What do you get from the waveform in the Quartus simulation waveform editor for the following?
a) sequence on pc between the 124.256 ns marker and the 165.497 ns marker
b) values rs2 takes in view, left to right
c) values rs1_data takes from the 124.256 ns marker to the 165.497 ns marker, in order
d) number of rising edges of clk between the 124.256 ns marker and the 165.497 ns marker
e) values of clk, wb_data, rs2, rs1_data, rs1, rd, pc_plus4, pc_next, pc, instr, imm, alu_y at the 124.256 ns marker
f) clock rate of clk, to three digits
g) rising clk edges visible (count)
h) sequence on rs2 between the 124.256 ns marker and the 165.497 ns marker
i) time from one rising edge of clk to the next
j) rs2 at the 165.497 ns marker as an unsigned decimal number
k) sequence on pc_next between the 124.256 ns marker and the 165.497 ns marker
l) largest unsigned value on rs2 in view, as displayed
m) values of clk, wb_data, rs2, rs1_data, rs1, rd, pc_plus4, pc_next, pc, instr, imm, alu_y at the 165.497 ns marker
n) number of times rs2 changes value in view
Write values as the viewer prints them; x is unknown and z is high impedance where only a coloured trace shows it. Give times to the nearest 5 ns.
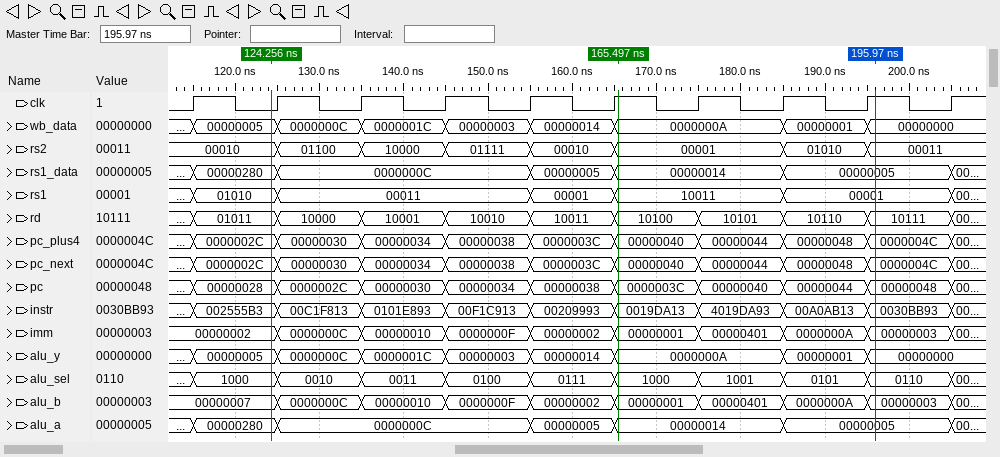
00000028, 0000002C, 00000030, 00000034, 00000038, 0000003C
00010, 01100, 10000, 01111, 00010, 00001, 01010, 00011
00000280, 0000000C, 00000005, 00000014
5
clk=0, wb_data=00000005, rs2=00010, rs1_data=00000280, rs1=01010, rd=01011, pc_plus4=0000002C, pc_next=0000002C, pc=00000028, instr=002555B3, imm=00000002, alu_y=00000005
100 MHz
10
00010, 01100, 10000, 01111, 00010, 00001
10 ns
1
0000002C, 00000030, 00000034, 00000038, 0000003C, 00000040
10000
clk=1, wb_data=0000000A, rs2=00001, rs1_data=00000014, rs1=10011, rd=10100, pc_plus4=00000040, pc_next=00000040, pc=0000003C, instr=0019DA13, imm=00000001, alu_y=0000000A
7
